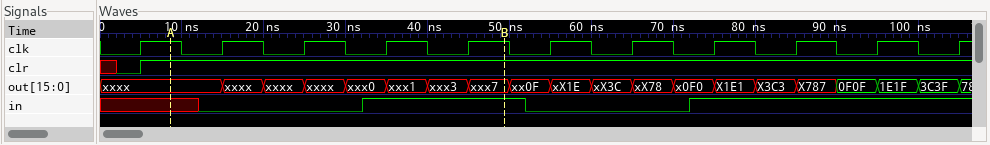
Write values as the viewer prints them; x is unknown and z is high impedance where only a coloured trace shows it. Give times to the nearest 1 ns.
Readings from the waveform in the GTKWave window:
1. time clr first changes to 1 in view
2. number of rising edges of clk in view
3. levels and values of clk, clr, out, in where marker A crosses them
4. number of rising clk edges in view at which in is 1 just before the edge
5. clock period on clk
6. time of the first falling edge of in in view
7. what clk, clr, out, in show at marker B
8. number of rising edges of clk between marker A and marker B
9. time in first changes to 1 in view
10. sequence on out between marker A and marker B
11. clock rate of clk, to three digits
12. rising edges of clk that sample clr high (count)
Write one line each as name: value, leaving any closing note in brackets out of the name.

time clr first changes to 1 in view: 5 ns
number of rising edges of clk in view: 11
levels and values of clk, clr, out, in where marker A crosses them: clk=1, clr=1, out=xxxx, in=x
number of rising clk edges in view at which in is 1 just before the edge: 6
clock period on clk: 10 ns
time of the first falling edge of in in view: 52 ns
what clk, clr, out, in show at marker B: clk=1, clr=1, out=xxx7, in=1
number of rising edges of clk between marker A and marker B: 4
time in first changes to 1 in view: 32 ns
sequence on out between marker A and marker B: xxxx, xxxx, xxxx, xxxx, xxx0, xxx1, xxx3, xxx7
clock rate of clk, to three digits: 100 MHz
rising edges of clk that sample clr high: 10
